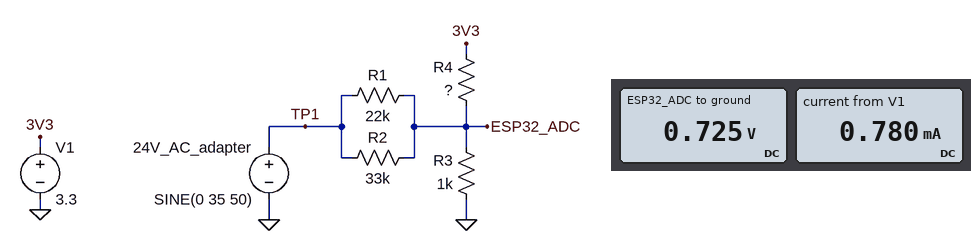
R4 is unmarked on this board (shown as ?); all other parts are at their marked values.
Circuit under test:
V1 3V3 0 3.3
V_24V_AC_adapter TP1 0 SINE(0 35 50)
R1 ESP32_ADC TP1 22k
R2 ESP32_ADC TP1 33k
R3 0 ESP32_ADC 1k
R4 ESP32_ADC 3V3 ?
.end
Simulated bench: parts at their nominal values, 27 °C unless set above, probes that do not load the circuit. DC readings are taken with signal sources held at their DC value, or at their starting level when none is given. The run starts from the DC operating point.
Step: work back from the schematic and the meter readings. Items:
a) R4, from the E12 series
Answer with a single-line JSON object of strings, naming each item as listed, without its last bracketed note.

{"R4, from the E12 series": "3.3 kΩ"}
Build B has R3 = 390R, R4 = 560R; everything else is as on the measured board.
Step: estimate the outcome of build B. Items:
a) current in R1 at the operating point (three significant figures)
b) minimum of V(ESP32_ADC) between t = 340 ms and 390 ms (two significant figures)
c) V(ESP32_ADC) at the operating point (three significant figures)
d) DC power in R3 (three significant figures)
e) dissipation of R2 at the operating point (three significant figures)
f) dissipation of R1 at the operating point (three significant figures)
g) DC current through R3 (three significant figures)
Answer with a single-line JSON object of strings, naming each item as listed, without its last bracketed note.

{"current in R1 at the operating point": "60.5 µA", "minimum of V(ESP32_ADC) between t = 340 ms and 390 ms": "730 mV", "V(ESP32_ADC) at the operating point": "1.33 V", "DC power in R3": "4.55 mW", "dissipation of R2 at the operating point": "53.7 µW", "dissipation of R1 at the operating point": "80.6 µW", "DC current through R3": "3.41 mA"}
